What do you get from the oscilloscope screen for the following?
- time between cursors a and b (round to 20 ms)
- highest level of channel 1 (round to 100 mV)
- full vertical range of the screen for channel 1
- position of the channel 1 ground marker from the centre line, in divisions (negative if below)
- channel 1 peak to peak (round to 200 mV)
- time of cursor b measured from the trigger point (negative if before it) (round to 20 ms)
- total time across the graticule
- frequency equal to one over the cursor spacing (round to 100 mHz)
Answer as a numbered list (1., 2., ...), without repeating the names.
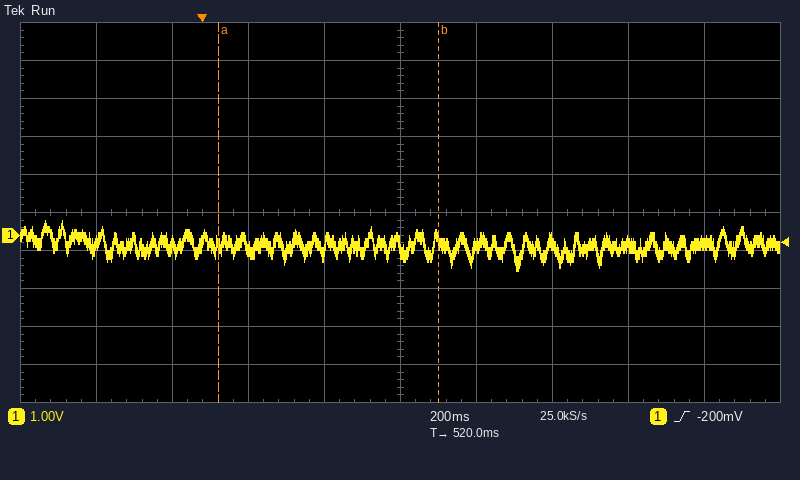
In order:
1. 580 ms
2. 400 mV
3. 10 V
4. -0.6 div
5. 1.4 V
6. +620 ms
7. 2 s
8. 1.7 Hz
